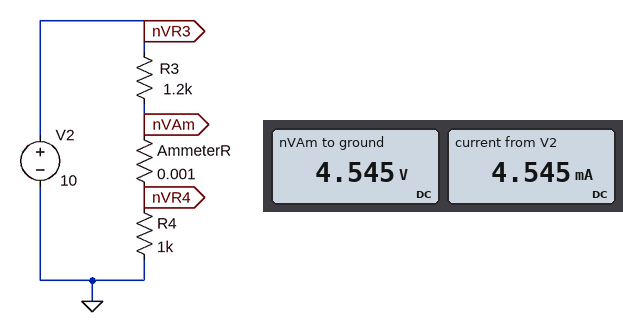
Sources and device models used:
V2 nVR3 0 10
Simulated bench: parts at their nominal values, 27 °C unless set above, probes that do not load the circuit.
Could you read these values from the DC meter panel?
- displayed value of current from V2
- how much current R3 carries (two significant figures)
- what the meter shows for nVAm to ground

4.545 mA
4.5 mA
4.545 V
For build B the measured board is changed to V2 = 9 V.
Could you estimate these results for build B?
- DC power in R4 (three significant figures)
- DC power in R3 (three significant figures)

16.7 mW
20.1 mW
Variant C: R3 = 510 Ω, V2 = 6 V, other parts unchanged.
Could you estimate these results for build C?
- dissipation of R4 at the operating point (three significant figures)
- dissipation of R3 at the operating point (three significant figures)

15.8 mW
8.05 mW
